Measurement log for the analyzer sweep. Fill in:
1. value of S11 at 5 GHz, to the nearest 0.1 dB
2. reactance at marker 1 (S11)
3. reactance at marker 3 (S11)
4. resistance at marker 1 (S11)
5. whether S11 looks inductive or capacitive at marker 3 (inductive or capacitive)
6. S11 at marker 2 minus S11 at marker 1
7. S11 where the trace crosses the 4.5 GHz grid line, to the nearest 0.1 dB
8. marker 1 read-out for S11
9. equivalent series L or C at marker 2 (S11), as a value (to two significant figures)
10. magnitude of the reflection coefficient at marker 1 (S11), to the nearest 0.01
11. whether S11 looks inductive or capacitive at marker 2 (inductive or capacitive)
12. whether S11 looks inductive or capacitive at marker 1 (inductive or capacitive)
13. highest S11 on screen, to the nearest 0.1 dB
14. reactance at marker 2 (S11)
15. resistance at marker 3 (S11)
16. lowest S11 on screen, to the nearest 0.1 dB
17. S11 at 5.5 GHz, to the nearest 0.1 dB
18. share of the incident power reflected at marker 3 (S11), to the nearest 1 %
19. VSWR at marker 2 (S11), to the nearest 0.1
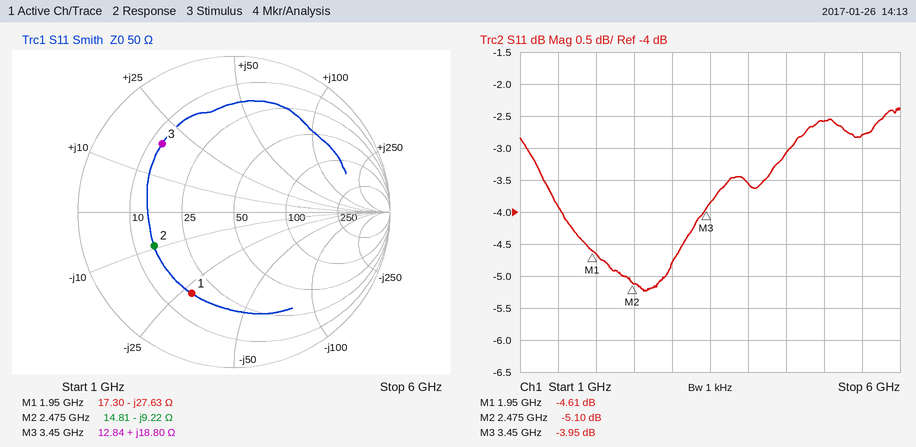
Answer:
-2.6 dB
-27.63 Ω
+18.80 Ω
17.30 Ω
inductive
-0.49 dB
-3.1 dB
-4.61 dB
7.0 pF
0.59
capacitive
capacitive
-2.4 dB
-9.22 Ω
12.84 Ω
-5.2 dB
-2.8 dB
40 %
3.5
